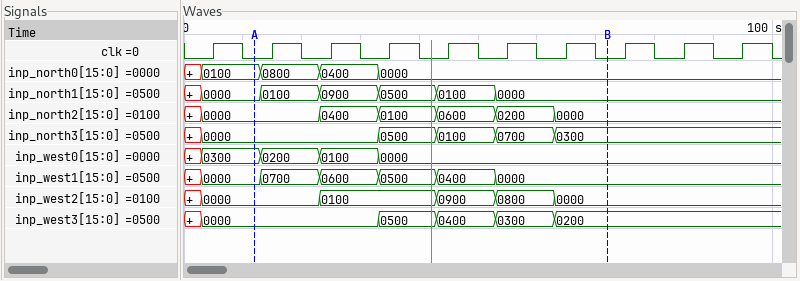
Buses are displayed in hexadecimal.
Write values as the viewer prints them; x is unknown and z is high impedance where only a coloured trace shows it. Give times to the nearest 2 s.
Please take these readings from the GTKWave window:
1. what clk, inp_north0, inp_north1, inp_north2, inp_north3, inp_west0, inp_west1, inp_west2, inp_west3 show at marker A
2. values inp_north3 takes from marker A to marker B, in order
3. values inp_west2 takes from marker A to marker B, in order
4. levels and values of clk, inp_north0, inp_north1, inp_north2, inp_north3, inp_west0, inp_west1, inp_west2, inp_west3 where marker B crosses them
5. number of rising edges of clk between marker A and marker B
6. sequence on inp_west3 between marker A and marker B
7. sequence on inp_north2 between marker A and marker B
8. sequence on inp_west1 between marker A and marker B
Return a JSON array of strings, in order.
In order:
["clk=0, inp_north0=0100, inp_north1=0000, inp_north2=0000, inp_north3=0000, inp_west0=0300, inp_west1=0000, inp_west2=0000, inp_west3=0000", "0000, 0500, 0100, 0700, 0300", "0000, 0100, 0900, 0800, 0000", "clk=0, inp_north0=0000, inp_north1=0000, inp_north2=0000, inp_north3=0300, inp_west0=0000, inp_west1=0000, inp_west2=0000, inp_west3=0200", "6", "0000, 0500, 0400, 0300, 0200", "0000, 0400, 0100, 0600, 0200, 0000", "0000, 0700, 0600, 0500, 0400, 0000"]
